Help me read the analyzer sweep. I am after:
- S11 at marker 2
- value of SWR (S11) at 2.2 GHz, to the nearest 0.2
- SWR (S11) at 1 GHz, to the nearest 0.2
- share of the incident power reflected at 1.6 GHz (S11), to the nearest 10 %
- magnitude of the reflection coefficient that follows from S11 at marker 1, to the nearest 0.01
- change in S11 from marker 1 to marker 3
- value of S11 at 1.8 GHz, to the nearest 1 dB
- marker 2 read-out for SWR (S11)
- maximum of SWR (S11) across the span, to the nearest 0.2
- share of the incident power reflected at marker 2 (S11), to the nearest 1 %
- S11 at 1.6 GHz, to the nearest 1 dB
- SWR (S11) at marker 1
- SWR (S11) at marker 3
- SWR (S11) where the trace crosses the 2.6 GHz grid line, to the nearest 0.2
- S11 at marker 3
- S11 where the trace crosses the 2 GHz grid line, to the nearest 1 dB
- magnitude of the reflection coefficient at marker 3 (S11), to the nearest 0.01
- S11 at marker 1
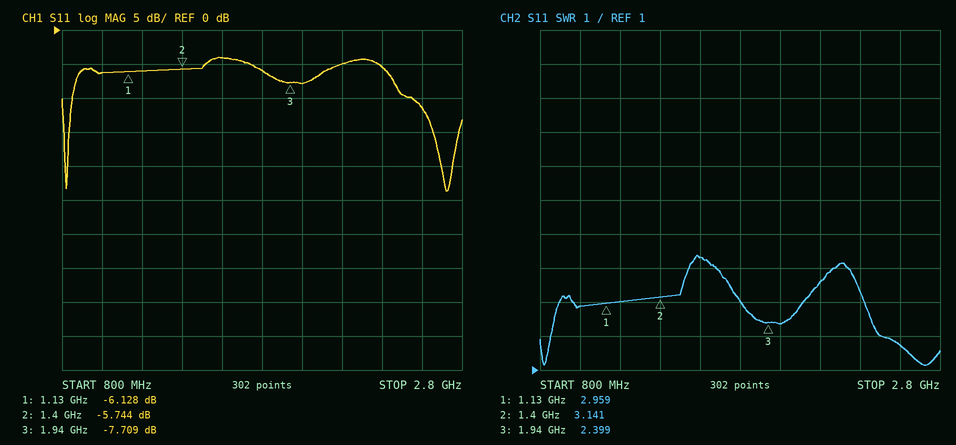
-5.744 dB
3.6
2.8
40 %
0.49
-1.581 dB
-6 dB
3.141
4.4
27 %
-4 dB
2.959
2.399
1.8
-7.709 dB
-8 dB
0.41
-6.128 dB
